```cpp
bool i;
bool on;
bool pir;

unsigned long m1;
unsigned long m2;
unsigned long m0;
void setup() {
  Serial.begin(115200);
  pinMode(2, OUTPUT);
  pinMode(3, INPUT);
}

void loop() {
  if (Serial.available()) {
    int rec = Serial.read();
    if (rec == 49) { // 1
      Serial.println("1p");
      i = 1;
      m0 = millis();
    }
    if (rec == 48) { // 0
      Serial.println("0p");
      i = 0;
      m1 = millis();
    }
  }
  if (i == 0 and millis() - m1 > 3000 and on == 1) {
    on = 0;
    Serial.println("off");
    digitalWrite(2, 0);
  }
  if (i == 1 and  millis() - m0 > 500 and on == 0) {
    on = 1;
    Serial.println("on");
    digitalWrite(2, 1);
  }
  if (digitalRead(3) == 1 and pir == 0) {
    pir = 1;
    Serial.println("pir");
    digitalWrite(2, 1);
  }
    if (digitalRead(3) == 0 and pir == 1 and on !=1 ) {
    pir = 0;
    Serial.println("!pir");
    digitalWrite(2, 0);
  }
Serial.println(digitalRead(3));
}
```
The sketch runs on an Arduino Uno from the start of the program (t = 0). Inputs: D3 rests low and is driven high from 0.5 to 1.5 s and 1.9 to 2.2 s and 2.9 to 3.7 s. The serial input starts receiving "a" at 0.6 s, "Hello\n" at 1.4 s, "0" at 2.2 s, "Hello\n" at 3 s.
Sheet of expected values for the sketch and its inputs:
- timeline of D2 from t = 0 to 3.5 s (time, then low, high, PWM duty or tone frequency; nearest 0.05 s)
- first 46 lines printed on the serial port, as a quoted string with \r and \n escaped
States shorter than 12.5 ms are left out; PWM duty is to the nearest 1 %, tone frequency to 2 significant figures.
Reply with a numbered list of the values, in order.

1. 0 s low; 0.5 s high; 1.5 s low; 1.9 s high; 2.2 s low; 2.9 s high
2. "0\r\n0\r\n0\r\n0\r\n0\r\n0\r\n0\r\n0\r\n0\r\n0\r\n0\r\n0\r\n0\r\n0\r\n0\r\n0\r\n0\r\n0\r\n0\r\n0\r\n0\r\n0\r\n0\r\n0\r\n0\r\n0\r\n0\r\n0\r\n0\r\n0\r\n0\r\n0\r\n0\r\n0\r\n0\r\n0\r\n0\r\n0\r\n0\r\n0\r\n0\r\n0\r\n0\r\n0\r\n0\r\n0\r\n"
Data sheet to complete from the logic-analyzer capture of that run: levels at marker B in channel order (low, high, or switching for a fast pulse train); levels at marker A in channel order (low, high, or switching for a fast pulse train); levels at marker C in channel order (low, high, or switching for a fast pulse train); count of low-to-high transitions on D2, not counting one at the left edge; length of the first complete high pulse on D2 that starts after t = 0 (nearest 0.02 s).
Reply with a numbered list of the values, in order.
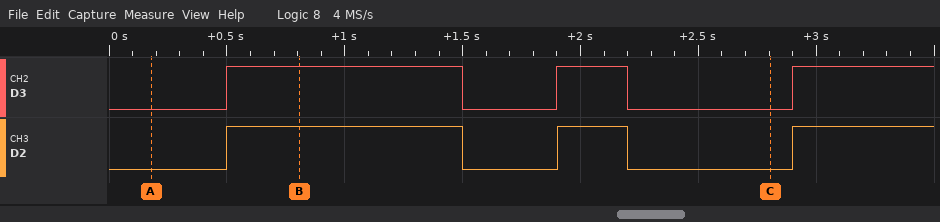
1. D3 high, D2 high
2. D3 low, D2 low
3. D3 low, D2 low
4. 3
5. 1.00 s
